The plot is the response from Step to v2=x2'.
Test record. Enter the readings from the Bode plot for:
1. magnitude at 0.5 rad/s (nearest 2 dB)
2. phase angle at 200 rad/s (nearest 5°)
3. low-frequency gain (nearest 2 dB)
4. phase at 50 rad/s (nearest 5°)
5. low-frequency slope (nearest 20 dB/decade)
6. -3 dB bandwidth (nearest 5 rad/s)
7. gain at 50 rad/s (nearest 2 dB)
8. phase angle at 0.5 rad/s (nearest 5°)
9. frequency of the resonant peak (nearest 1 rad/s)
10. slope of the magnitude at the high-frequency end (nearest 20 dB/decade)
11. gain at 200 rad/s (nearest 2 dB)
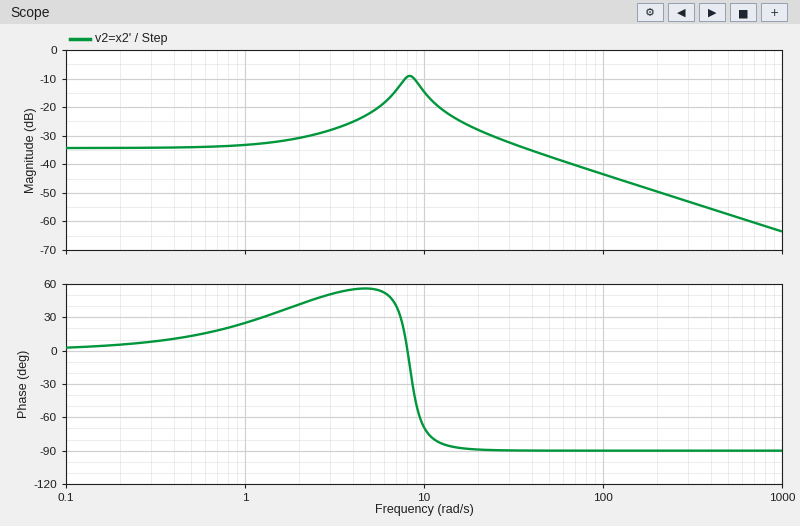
-34 dB
-90°
-34 dB
-90°
0 dB/decade
50 rad/s
-38 dB
15°
8 rad/s
-20 dB/decade
-50 dB
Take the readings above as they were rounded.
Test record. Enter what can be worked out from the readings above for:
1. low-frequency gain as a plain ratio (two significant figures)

0.020
